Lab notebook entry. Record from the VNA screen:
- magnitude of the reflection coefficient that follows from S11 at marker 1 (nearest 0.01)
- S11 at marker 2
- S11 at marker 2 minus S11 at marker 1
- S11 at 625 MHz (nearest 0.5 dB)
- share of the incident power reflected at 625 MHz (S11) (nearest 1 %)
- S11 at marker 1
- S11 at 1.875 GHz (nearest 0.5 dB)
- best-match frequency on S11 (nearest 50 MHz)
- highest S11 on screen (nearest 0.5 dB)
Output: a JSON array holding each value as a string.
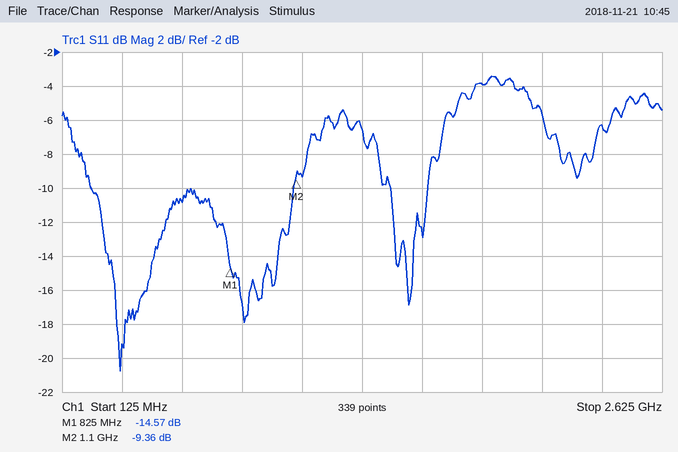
["0.19", "-9.36 dB", "5.21 dB", "-11.0 dB", "8 %", "-14.57 dB", "-4.0 dB", "350 MHz", "-3.5 dB"]
